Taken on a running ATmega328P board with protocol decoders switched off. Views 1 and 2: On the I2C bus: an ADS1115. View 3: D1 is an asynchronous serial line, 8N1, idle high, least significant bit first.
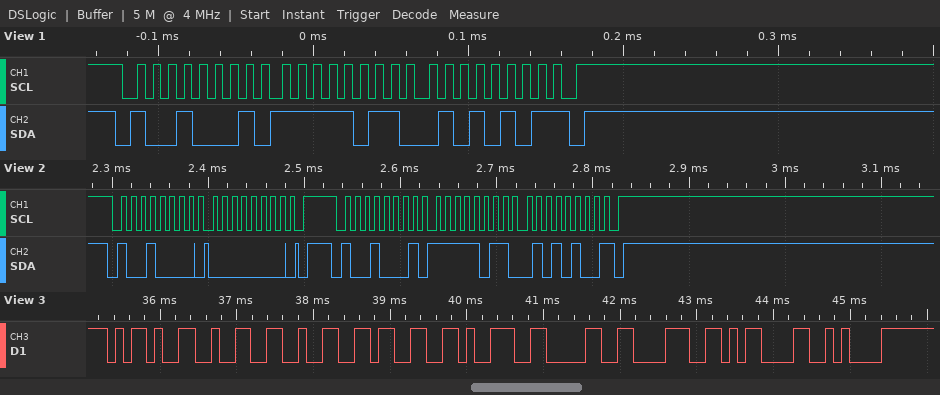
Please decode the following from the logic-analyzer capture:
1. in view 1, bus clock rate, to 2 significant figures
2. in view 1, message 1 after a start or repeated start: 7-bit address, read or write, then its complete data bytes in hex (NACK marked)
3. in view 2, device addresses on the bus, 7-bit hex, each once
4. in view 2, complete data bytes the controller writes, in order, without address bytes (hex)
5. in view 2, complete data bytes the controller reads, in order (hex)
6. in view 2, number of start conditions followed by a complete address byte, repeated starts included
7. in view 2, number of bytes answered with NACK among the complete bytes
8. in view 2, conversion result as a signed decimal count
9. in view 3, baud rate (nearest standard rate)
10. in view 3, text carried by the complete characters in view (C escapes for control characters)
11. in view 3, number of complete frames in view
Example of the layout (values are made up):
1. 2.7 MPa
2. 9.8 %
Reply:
1. 100 kHz
2. 0x48 read: FB 55 NACK
3. 0x48
4. 00
5. FB 54
6. 2
7. 1
8. -1196
9. 9600 baud
10. "-223908\r\n"
11. 9
